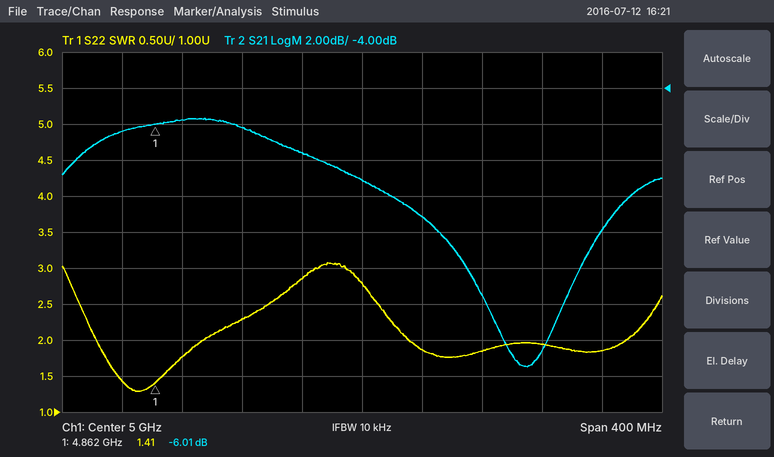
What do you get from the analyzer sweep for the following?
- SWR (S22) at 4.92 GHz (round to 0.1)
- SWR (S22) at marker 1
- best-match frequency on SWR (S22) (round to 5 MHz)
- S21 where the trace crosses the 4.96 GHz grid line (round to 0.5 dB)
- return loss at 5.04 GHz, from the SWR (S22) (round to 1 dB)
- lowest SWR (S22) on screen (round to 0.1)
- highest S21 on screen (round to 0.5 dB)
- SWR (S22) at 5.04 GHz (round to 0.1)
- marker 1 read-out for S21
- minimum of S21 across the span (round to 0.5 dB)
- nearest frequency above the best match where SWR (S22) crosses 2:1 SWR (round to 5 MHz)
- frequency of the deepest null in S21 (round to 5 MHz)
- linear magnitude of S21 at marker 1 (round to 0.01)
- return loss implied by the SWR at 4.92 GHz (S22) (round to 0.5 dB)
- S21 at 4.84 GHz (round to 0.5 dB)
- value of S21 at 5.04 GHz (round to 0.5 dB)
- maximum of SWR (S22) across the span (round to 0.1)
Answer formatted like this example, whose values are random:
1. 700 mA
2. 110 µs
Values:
1. 2.3
2. 1.41
3. 4.850 GHz
4. -7.5 dB
5. 10 dB
6. 1.3
7. -5.5 dB
8. 1.9
9. -6.01 dB
10. -19.5 dB
11. 4.895 GHz
12. 5.110 GHz
13. 0.50
14. 8.0 dB
15. -6.5 dB
16. -11.0 dB
17. 3.1
